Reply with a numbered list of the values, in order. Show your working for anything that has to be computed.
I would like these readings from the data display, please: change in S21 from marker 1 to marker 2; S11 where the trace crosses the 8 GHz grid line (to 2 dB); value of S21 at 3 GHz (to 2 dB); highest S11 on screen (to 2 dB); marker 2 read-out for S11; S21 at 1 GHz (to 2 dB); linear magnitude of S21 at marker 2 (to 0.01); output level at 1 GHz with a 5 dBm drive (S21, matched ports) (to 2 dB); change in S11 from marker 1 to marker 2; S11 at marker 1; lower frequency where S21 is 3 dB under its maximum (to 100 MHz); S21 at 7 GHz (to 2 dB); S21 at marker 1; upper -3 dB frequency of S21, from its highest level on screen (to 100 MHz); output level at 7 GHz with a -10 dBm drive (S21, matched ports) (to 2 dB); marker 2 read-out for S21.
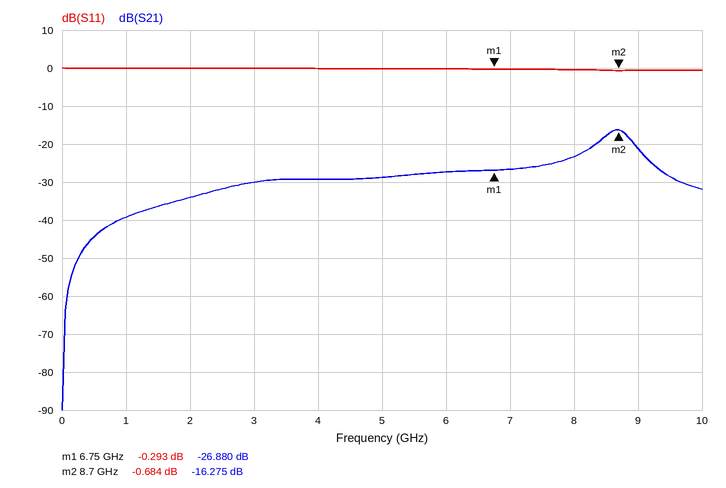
1. -16.275 − (-26.88) = 10.605 dB
2. 0 dB
3. -30 dB
4. 0 dB
5. -0.684 dB
6. -40 dB
7. 10^(-16.275/20) ≈ 0.15
8. 5 dBm + (-40 dB) = -34 dBm
9. -0.684 − (-0.293) = -0.391 dB
10. -0.293 dB
11. 8.4 GHz
12. -26 dB
13. -26.880 dB
14. 8.9 GHz
15. -10 dBm + (-26 dB) = -36 dBm
16. -16.275 dB
